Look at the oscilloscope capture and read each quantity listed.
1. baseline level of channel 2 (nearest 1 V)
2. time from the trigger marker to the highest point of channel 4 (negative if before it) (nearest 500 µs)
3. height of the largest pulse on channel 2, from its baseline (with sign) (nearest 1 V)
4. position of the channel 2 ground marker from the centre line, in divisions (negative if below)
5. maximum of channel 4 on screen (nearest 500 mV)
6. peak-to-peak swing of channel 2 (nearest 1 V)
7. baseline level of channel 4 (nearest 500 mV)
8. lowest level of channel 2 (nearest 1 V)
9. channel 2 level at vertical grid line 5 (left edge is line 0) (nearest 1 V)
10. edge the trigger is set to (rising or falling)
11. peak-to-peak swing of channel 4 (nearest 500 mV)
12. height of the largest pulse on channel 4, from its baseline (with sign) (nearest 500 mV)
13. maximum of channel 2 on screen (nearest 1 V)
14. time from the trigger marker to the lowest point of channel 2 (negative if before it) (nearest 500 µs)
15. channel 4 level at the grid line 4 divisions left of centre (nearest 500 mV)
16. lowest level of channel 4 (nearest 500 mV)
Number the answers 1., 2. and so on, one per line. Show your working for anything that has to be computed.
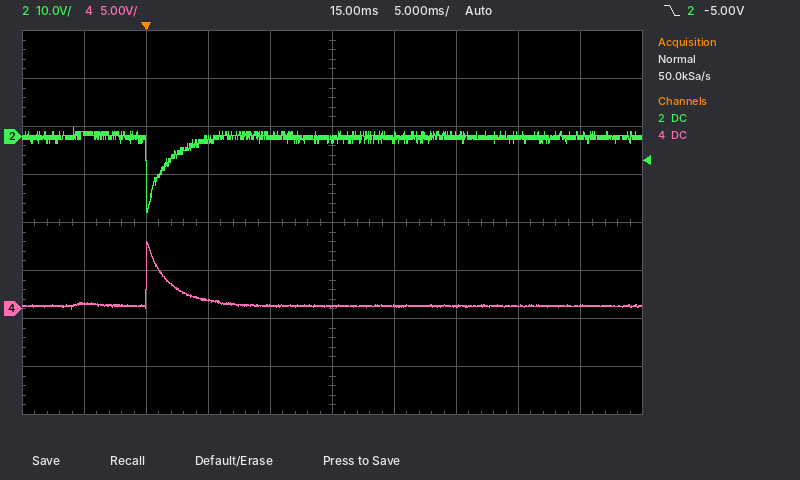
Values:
1. 0 V
2. 0.0 ms
3. -16 V − (0 V) = -16 V
4. +1.8 div
5. 7.0 V
6. 2 V − (-16 V) = 18 V
7. 500 mV
8. -16 V
9. -1 V
10. falling
11. 7.0 V − (0.0 V) = 7.0 V
12. 7.0 V − (500 mV) = +6.5 V
13. 2 V
14. 0.0 ms
15. 500 mV
16. 0.0 V
